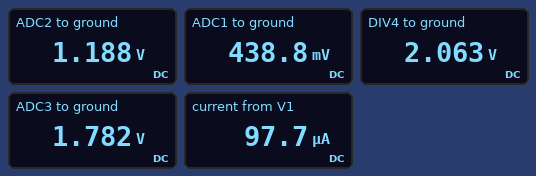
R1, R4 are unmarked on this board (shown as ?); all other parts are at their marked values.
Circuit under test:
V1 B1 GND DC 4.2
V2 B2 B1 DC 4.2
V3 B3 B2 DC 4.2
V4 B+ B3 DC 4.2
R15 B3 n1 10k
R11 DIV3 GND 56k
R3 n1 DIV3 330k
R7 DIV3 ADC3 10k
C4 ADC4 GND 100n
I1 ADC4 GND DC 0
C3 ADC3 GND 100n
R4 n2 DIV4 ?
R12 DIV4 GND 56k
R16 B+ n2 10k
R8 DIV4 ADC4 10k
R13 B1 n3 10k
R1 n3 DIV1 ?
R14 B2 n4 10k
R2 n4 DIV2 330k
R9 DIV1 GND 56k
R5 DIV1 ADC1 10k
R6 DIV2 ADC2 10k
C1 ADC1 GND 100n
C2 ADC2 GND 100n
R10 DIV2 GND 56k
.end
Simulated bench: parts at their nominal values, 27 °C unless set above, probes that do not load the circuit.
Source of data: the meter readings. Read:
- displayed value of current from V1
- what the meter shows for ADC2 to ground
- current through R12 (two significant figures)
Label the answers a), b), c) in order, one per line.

a) 97.7 µA
b) 1.188 V
c) 37 µA
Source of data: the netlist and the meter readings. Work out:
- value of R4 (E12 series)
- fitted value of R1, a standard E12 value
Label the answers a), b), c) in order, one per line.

a) 390 kΩ
b) 470 kΩ
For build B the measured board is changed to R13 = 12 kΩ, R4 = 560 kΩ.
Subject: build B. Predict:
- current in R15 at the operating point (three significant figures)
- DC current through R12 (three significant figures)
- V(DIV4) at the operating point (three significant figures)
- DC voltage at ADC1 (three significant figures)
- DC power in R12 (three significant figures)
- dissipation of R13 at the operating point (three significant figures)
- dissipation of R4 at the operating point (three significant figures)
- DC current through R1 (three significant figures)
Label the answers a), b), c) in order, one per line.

a) 31.8 µA
b) 26.8 µA
c) 1.50 V
d) 437 mV
e) 40.3 µW
f) 731 nW
g) 403 µW
h) 7.81 µA
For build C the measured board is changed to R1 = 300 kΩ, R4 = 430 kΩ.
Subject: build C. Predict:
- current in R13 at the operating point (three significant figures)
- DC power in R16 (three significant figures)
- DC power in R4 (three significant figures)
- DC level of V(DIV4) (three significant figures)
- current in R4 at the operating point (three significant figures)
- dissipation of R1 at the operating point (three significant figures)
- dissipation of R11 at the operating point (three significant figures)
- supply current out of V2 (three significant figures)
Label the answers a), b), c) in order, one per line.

a) 11.5 µA
b) 11.5 µW
c) 493 µW
d) 1.90 V
e) 33.9 µA
f) 39.5 µW
g) 56.7 µW
h) 86.9 µA
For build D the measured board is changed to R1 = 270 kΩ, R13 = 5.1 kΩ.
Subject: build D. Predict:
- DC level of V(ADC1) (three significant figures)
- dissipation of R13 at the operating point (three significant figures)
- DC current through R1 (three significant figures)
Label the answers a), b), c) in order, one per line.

a) 710 mV
b) 821 nW
c) 12.7 µA
